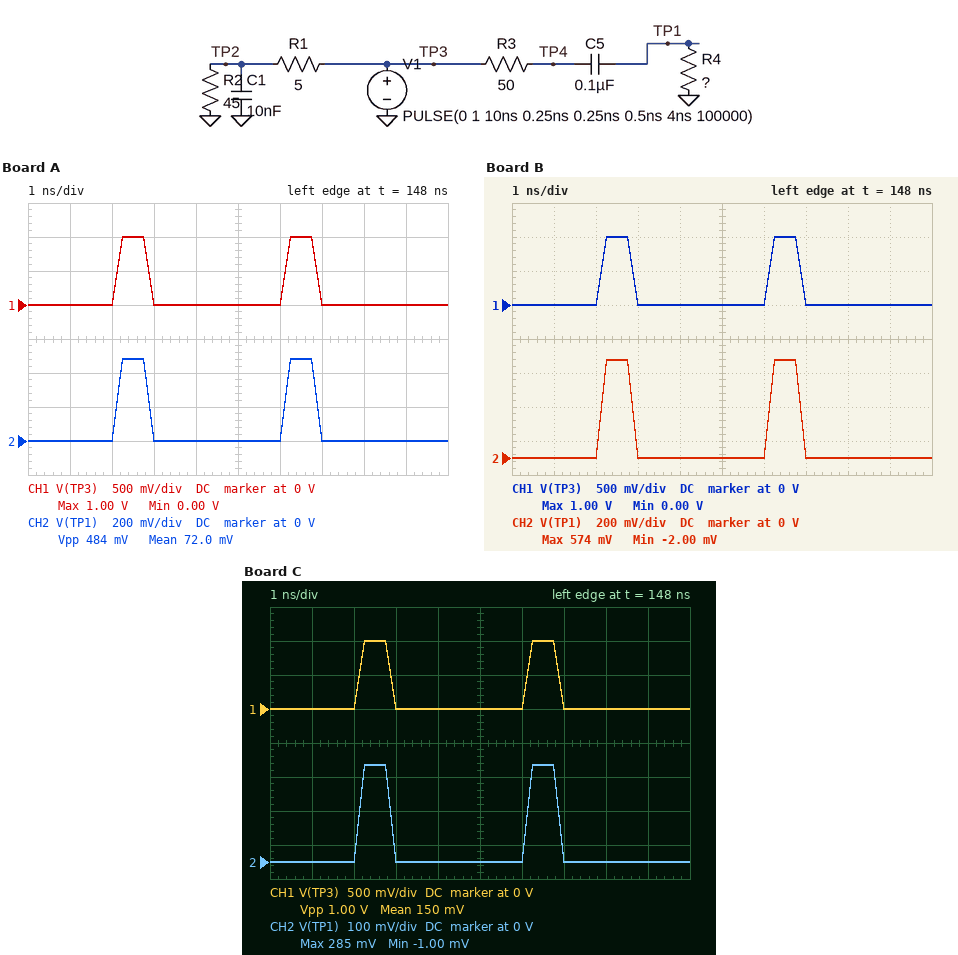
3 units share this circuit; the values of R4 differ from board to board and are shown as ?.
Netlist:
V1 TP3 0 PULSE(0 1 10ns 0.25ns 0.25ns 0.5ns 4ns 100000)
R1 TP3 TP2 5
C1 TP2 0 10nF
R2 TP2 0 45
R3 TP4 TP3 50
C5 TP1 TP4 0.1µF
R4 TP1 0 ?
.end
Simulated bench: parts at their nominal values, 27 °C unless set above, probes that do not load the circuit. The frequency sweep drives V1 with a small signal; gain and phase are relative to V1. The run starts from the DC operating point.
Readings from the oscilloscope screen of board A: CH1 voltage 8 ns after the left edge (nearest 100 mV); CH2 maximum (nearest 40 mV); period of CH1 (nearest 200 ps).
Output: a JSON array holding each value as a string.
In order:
["0 V", "480 mV", "4.0 ns"]
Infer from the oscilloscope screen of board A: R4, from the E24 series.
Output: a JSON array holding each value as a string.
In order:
["47 Ω"]
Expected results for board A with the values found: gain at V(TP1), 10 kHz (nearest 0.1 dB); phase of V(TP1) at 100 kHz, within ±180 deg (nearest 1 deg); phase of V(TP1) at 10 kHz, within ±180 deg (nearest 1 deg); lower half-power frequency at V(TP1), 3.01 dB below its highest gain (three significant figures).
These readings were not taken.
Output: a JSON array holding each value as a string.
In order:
["-12.0 dB", "9 deg", "59 deg", "16.4 kHz"]
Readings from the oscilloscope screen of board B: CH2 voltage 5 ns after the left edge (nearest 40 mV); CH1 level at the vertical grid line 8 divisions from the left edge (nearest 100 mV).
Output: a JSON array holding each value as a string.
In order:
["0 V", "0 V"]
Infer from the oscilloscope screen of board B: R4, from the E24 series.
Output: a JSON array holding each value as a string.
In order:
["68 Ω"]
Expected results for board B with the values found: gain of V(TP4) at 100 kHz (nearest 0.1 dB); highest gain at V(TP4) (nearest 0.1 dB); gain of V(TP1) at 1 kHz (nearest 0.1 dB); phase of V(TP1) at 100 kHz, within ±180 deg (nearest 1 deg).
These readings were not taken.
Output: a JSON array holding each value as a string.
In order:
["-4.6 dB", "0 dB", "-27.4 dB", "8 deg"]
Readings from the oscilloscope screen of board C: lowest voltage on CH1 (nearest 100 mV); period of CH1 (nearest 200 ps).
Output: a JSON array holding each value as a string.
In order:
["0 V", "4.0 ns"]
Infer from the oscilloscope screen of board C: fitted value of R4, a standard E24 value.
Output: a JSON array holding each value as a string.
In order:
["20 Ω"]
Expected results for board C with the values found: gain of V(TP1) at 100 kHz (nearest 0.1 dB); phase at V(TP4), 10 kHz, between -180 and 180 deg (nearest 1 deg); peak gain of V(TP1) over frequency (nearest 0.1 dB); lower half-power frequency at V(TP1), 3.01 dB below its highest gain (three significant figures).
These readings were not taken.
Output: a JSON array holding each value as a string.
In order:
["-11.1 dB", "-17 deg", "-10.9 dB", "22.7 kHz"]
